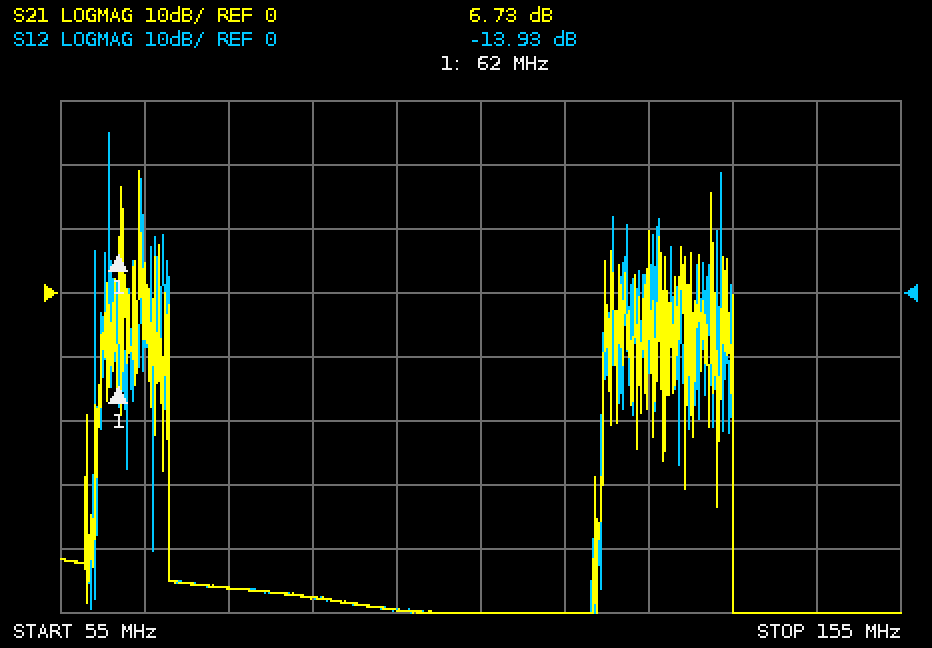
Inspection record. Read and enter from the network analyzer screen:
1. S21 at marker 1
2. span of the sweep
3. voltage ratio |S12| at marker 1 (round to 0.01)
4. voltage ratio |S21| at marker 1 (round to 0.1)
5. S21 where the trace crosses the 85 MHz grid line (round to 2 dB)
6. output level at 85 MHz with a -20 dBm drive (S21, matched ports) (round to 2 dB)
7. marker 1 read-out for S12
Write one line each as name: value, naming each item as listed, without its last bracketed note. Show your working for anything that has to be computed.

S21 at marker 1: 6.73 dB
span of the sweep: 100 MHz
voltage ratio |S12| at marker 1: 10^(-13.93/20) ≈ 0.20
voltage ratio |S21| at marker 1: 10^(6.73/20) ≈ 2.2
S21 where the trace crosses the 85 MHz grid line: -48 dB
output level at 85 MHz with a -20 dBm drive (S21, matched ports): -20 dBm + (-48 dB) = -68 dBm
marker 1 read-out for S12: -13.93 dB
